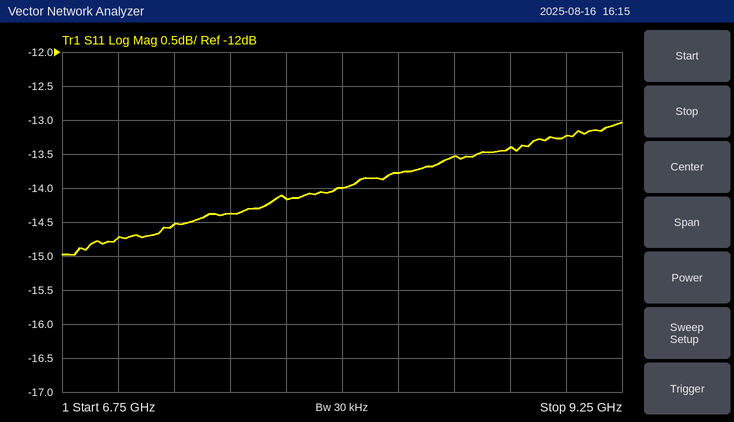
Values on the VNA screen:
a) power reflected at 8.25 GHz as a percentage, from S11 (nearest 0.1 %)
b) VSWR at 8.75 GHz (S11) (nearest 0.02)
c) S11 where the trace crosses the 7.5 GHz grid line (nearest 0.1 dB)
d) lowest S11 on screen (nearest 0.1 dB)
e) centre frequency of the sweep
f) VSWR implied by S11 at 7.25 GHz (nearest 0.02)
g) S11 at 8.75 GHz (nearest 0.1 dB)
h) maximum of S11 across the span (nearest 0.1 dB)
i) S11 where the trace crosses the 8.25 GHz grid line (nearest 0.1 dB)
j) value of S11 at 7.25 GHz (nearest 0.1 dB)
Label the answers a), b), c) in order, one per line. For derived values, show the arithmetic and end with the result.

a) 10^(-13.8/10) ≈ 4.2 %
b) |Γ| = 10^(-13.4/20) = 0.2138; VSWR = (1 + 0.2138)/(1 − 0.2138) ≈ 1.54
c) -14.4 dB
d) -15.0 dB
e) 8 GHz
f) |Γ| = 10^(-14.5/20) = 0.1884; VSWR = (1 + 0.1884)/(1 − 0.1884) ≈ 1.46
g) -13.4 dB
h) -13.0 dB
i) -13.8 dB
j) -14.5 dB
